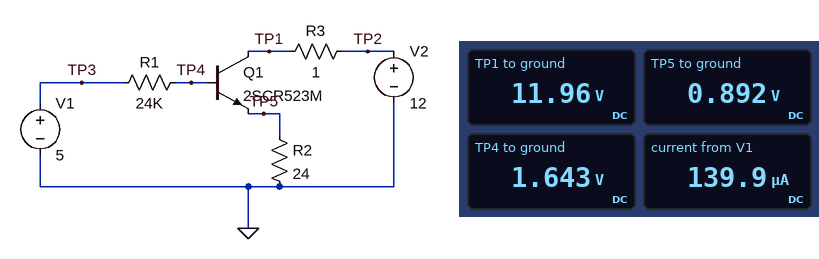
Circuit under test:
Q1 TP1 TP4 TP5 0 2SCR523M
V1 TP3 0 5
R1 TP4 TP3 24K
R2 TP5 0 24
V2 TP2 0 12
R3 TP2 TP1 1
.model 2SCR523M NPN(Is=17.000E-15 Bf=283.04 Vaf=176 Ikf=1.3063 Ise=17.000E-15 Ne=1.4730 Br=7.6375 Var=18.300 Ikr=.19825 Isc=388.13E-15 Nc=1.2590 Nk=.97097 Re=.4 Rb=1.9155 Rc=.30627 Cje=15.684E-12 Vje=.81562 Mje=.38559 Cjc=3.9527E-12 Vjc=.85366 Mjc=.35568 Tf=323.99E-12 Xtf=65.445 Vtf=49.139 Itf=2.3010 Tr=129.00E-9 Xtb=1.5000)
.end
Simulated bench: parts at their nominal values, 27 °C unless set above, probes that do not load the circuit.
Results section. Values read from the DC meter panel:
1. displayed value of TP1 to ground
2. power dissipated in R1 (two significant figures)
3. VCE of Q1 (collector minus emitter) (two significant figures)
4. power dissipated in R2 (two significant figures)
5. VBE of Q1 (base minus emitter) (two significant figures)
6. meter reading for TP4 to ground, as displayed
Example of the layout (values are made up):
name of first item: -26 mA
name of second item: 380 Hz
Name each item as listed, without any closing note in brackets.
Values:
displayed value of TP1 to ground: 11.96 V
power dissipated in R1: 470 µW
VCE of Q1 (collector minus emitter): 11 V
power dissipated in R2: 33 mW
VBE of Q1 (base minus emitter): 750 mV
meter reading for TP4 to ground, as displayed: 1.643 V
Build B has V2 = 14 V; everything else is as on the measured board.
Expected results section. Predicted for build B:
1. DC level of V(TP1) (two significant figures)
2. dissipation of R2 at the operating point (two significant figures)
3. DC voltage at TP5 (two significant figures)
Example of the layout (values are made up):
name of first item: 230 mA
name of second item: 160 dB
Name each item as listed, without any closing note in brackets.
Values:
DC level of V(TP1): 14 V
dissipation of R2 at the operating point: 34 mW
DC voltage at TP5: 900 mV
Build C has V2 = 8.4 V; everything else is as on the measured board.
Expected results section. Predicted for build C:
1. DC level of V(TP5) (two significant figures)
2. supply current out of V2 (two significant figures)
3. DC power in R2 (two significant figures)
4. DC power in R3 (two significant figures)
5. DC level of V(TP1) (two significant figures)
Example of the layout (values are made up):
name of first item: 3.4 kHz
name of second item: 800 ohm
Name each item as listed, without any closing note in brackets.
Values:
DC level of V(TP5): 880 mV
supply current out of V2: 36 mA
DC power in R2: 32 mW
DC power in R3: 1.3 mW
DC level of V(TP1): 8.4 V
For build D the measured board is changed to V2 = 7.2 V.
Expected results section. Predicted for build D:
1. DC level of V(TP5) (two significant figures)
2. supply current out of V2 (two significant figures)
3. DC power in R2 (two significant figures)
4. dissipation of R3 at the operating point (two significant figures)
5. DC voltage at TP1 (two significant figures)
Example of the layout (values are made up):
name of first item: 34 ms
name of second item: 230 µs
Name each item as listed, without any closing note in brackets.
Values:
DC level of V(TP5): 870 mV
supply current out of V2: 36 mA
DC power in R2: 32 mW
dissipation of R3 at the operating point: 1.3 mW
DC voltage at TP1: 7.2 V
